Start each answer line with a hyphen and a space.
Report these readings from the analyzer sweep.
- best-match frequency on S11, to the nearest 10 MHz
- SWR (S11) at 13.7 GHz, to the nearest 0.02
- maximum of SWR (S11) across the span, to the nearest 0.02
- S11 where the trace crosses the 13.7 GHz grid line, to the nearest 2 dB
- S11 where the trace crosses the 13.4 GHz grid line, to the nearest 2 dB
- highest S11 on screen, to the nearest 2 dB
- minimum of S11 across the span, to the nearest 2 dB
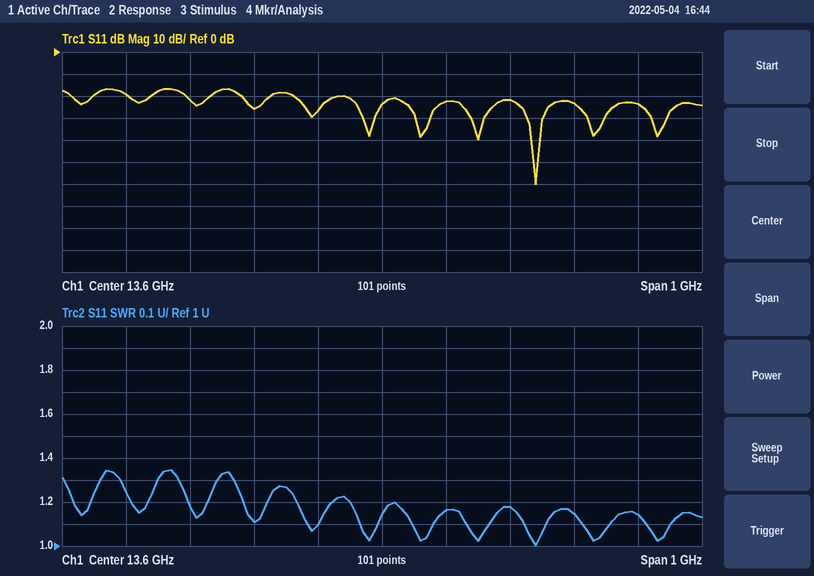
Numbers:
- 13.84 GHz
- 1.16
- 1.34
- -22 dB
- -26 dB
- -16 dB
- -60 dB
